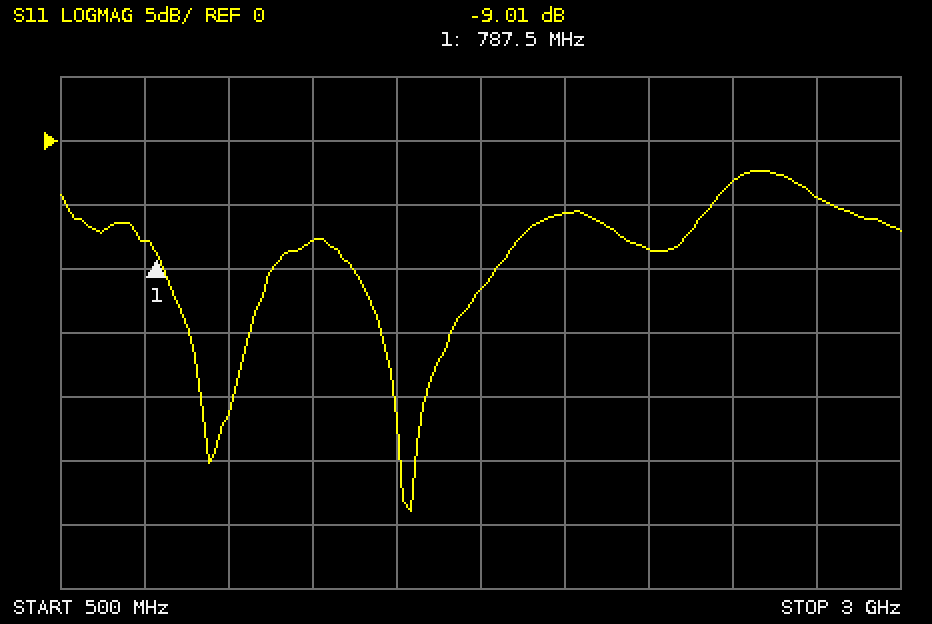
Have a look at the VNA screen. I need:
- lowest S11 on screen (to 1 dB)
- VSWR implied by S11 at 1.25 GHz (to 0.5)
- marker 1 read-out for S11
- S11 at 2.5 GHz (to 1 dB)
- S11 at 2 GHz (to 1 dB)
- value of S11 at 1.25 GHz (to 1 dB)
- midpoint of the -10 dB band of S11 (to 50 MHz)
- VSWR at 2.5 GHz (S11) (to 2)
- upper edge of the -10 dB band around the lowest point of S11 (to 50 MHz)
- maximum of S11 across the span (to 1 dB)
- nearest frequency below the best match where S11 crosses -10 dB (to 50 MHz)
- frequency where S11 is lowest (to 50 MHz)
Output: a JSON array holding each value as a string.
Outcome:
["-29 dB", "2.5", "-9.01 dB", "-3 dB", "-6 dB", "-8 dB", "1.60 GHz", "6", "1.80 GHz", "-2 dB", "1.35 GHz", "1.55 GHz"]
